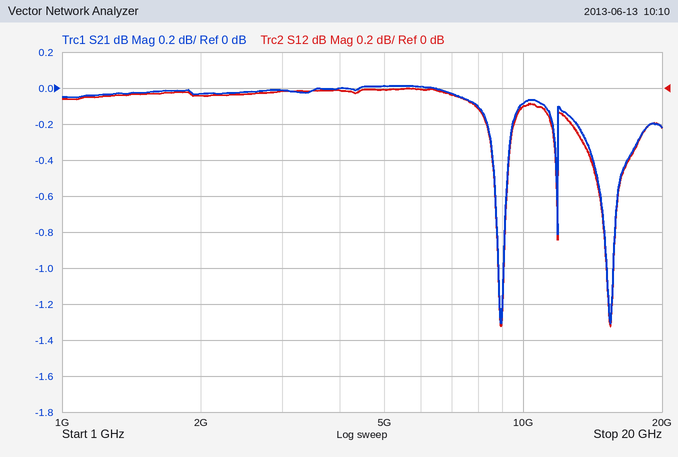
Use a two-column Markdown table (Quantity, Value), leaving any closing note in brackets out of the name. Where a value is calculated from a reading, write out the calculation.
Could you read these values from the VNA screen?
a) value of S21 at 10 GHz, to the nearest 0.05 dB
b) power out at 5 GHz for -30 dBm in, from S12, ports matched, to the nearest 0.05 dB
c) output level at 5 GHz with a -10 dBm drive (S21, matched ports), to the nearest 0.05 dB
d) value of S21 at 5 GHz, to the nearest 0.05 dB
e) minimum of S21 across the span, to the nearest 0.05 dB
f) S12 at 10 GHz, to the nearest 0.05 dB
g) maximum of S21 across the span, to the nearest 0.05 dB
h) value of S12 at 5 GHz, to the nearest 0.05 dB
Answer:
| Quantity | Value |
|---|---|
| value of S21 at 10 GHz, to the nearest 0.05 dB | -0.10 dB |
| power out at 5 GHz for -30 dBm in, from S12, ports matched, to the nearest 0.05 dB | -30 dBm + (0.00 dB) = -30.00 dBm |
| output level at 5 GHz with a -10 dBm drive (S21, matched ports), to the nearest 0.05 dB | -10 dBm + (0.00 dB) = -10.00 dBm |
| value of S21 at 5 GHz, to the nearest 0.05 dB | 0.00 dB |
| minimum of S21 across the span, to the nearest 0.05 dB | -1.30 dB |
| S12 at 10 GHz, to the nearest 0.05 dB | -0.10 dB |
| maximum of S21 across the span, to the nearest 0.05 dB | 0.00 dB |
| value of S12 at 5 GHz, to the nearest 0.05 dB | 0.00 dB |
